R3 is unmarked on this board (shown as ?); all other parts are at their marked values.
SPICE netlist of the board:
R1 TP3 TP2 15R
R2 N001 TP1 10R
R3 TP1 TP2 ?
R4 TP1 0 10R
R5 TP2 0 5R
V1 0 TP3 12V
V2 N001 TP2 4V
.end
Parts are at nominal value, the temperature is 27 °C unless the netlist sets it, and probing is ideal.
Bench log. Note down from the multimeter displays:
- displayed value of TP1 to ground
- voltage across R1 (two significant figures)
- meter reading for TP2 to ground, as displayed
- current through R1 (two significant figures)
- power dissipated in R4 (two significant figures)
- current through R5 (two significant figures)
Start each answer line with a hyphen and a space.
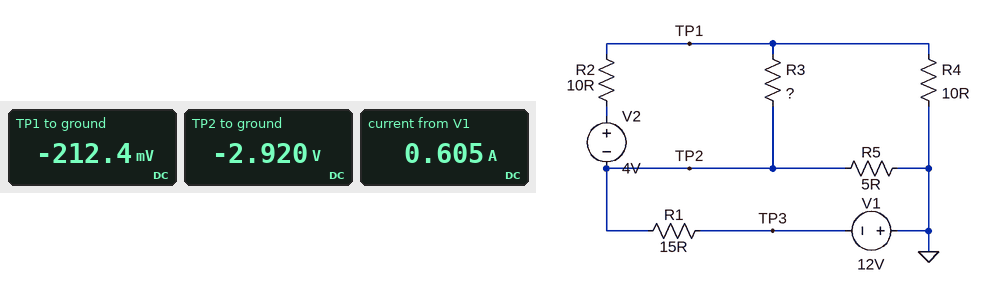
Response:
- -212.4 mV
- 9.1 V
- -2.920 V
- 610 mA
- 4.5 mW
- 580 mA
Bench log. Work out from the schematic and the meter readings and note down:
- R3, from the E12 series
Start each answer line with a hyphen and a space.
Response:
- 18 Ω
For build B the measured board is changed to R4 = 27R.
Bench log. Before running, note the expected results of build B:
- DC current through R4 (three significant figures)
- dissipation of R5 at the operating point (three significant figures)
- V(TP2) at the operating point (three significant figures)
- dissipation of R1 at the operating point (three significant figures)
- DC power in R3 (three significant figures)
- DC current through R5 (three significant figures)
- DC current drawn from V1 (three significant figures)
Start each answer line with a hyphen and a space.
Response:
- 11.5 mA
- 1.75 W
- -2.96 V
- 5.45 W
- 389 mW
- 591 mA
- 603 mA
